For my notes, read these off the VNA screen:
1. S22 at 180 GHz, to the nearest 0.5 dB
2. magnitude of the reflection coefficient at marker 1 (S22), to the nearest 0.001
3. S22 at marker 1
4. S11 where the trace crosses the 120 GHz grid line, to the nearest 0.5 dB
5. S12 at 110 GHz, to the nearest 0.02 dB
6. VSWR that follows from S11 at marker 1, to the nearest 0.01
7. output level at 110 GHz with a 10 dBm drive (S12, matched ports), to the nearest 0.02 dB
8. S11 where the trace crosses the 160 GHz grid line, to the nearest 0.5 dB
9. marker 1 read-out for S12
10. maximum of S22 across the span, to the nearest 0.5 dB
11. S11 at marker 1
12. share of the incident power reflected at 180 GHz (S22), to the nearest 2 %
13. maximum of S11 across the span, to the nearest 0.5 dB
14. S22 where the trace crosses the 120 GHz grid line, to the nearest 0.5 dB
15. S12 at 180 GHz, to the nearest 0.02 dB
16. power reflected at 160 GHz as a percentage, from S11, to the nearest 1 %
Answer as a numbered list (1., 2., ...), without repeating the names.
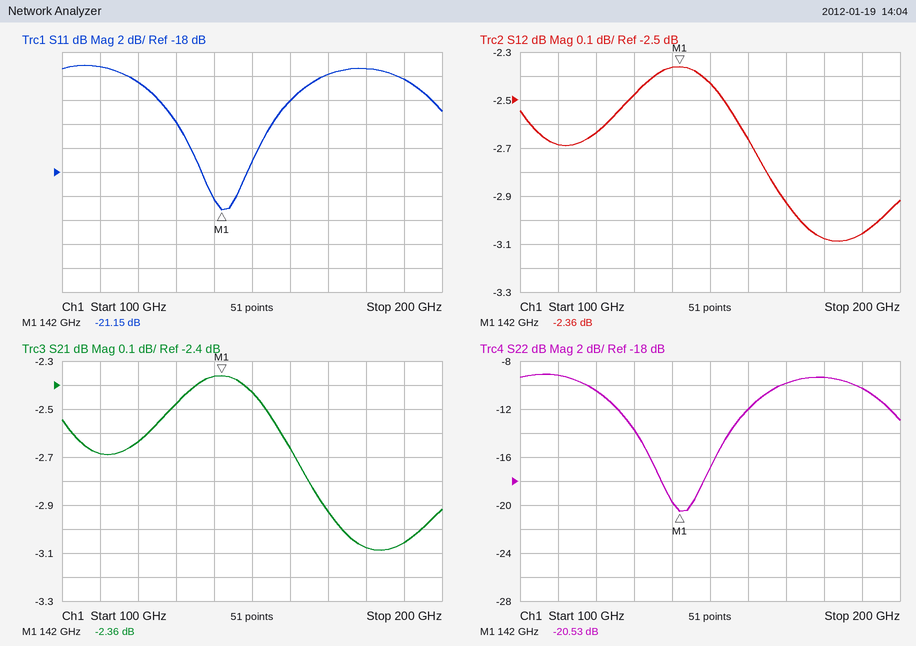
1. -9.5 dB
2. 0.094
3. -20.53 dB
4. -10.5 dB
5. -2.68 dB
6. 1.19
7. 7.32 dBm
8. -12.0 dB
9. -2.36 dB
10. -9.0 dB
11. -21.15 dB
12. 12 %
13. -9.0 dB
14. -10.5 dB
15. -3.08 dB
16. 6 %
